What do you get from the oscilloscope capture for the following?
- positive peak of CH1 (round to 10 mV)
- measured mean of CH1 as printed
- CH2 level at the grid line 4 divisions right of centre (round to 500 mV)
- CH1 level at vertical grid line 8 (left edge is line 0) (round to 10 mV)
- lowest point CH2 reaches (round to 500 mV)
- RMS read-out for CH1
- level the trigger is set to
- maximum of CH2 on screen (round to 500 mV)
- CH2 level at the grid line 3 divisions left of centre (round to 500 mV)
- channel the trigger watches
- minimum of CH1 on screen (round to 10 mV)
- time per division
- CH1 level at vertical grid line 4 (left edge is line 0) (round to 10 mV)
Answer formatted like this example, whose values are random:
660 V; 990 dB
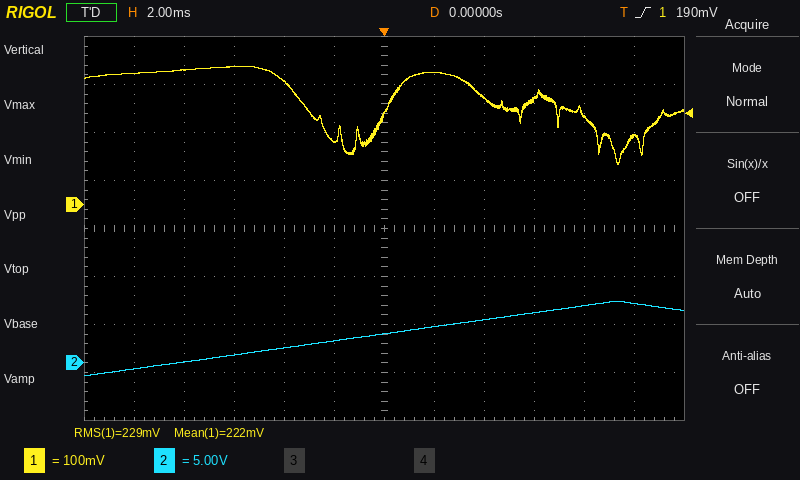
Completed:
290 mV; 222 mV; 6.0 V; 220 mV; -1.5 V; 229 mV; 190 mV; 6.5 V; 1.0 V; CH1; 80 mV; 2 ms; 260 mV
